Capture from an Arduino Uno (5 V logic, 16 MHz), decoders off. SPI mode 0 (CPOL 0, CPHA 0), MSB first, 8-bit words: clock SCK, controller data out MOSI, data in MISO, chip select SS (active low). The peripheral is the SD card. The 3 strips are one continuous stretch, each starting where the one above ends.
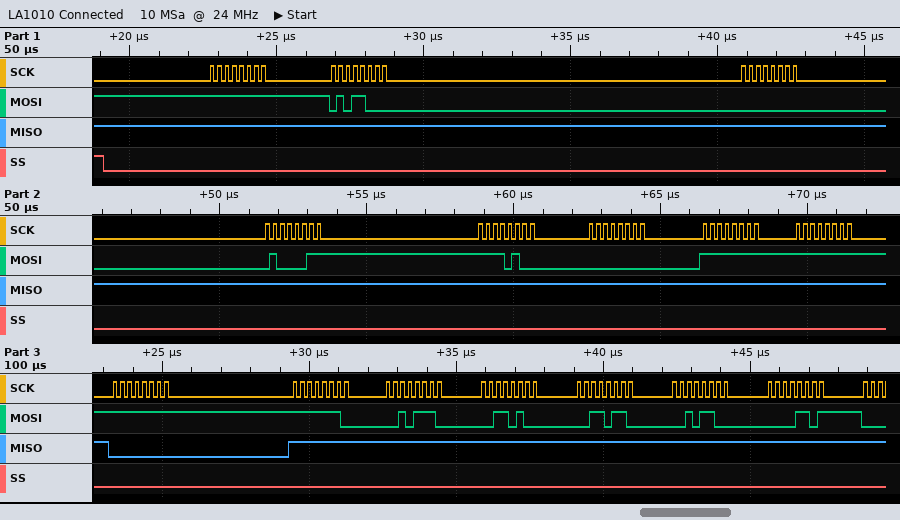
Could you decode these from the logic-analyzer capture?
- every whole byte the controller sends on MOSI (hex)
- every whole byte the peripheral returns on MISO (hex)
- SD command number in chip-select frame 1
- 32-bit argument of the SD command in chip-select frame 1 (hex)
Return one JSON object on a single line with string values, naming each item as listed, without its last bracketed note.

{"every whole byte the controller sends on MOSI": "FF 58 00 43 F4 00 FF FF FF FE 2E 34 36 2C 0D", "every whole byte the peripheral returns on MISO": "FF FF FF FF FF FF FF FF 00 FF FF FF FF FF FF", "SD command number in chip-select frame 1": "CMD24", "32-bit argument of the SD command in chip-select frame 1": "0x0043F400"}
